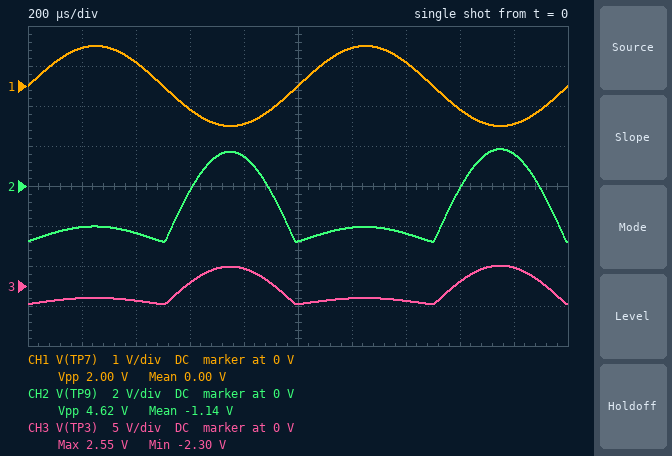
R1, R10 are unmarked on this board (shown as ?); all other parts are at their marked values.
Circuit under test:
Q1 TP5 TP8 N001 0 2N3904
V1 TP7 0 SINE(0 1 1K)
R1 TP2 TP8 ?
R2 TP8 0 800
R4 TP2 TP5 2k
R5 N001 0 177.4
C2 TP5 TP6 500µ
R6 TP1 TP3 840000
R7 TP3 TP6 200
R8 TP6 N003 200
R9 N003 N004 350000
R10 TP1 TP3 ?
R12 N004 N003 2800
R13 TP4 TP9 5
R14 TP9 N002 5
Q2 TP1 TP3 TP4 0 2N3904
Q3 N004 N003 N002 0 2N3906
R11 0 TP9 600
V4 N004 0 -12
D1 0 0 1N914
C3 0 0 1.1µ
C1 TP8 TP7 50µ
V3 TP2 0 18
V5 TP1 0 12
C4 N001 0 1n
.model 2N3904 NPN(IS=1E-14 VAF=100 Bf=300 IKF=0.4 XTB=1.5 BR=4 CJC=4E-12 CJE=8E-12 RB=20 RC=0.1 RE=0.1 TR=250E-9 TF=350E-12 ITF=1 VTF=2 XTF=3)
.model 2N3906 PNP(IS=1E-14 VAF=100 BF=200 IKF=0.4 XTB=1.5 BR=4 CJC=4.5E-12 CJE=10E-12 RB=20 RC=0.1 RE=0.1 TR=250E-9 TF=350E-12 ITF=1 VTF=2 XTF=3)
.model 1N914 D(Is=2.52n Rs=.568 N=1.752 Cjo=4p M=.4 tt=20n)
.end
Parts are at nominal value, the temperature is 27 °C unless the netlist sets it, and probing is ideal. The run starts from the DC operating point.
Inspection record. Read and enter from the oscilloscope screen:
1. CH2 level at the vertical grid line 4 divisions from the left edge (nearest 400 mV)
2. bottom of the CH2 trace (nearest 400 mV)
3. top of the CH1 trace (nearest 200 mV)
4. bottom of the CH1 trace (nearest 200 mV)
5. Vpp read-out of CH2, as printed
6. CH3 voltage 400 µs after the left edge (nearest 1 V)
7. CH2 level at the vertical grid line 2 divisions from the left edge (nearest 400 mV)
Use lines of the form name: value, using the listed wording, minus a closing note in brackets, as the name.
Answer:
CH2 level at the vertical grid line 4 divisions from the left edge: 1.6 V
bottom of the CH2 trace: -2.8 V
top of the CH1 trace: 1.0 V
bottom of the CH1 trace: -1.0 V
Vpp read-out of CH2, as printed: 4.62 V
CH3 voltage 400 µs after the left edge: -2 V
CH2 level at the vertical grid line 2 divisions from the left edge: -2.4 V
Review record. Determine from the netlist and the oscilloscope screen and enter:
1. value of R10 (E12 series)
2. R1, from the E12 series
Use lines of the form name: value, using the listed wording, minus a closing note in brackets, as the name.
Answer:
value of R10: 4.7 kΩ
R1, from the E12 series: 4.7 kΩ
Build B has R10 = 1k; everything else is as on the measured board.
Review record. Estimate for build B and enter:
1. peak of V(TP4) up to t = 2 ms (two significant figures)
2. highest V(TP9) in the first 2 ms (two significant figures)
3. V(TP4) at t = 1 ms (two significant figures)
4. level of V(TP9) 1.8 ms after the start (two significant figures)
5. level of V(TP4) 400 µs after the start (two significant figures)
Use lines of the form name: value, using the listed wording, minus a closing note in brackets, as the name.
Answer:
peak of V(TP4) up to t = 2 ms: 8.1 V
highest V(TP9) in the first 2 ms: 7.9 V
V(TP4) at t = 1 ms: 5.5 V
level of V(TP9) 1.8 ms after the start: 7.7 V
level of V(TP4) 400 µs after the start: 5.8 V
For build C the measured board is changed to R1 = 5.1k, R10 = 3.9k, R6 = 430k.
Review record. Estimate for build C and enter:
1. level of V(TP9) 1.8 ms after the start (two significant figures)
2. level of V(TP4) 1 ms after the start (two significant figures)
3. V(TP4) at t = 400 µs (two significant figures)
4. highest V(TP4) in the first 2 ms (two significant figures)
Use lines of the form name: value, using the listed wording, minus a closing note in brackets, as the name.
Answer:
level of V(TP9) 1.8 ms after the start: 2.7 V
level of V(TP4) 1 ms after the start: -1.8 V
V(TP4) at t = 400 µs: -1.4 V
highest V(TP4) in the first 2 ms: 2.9 V
